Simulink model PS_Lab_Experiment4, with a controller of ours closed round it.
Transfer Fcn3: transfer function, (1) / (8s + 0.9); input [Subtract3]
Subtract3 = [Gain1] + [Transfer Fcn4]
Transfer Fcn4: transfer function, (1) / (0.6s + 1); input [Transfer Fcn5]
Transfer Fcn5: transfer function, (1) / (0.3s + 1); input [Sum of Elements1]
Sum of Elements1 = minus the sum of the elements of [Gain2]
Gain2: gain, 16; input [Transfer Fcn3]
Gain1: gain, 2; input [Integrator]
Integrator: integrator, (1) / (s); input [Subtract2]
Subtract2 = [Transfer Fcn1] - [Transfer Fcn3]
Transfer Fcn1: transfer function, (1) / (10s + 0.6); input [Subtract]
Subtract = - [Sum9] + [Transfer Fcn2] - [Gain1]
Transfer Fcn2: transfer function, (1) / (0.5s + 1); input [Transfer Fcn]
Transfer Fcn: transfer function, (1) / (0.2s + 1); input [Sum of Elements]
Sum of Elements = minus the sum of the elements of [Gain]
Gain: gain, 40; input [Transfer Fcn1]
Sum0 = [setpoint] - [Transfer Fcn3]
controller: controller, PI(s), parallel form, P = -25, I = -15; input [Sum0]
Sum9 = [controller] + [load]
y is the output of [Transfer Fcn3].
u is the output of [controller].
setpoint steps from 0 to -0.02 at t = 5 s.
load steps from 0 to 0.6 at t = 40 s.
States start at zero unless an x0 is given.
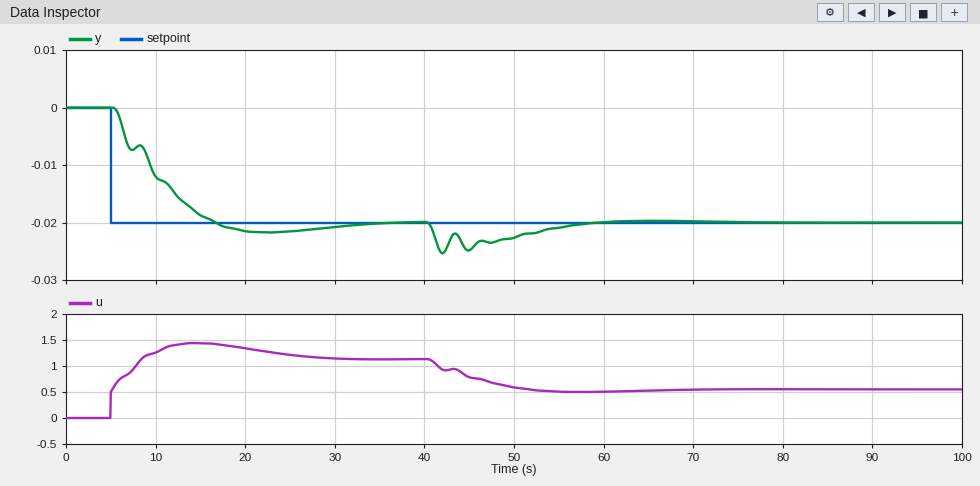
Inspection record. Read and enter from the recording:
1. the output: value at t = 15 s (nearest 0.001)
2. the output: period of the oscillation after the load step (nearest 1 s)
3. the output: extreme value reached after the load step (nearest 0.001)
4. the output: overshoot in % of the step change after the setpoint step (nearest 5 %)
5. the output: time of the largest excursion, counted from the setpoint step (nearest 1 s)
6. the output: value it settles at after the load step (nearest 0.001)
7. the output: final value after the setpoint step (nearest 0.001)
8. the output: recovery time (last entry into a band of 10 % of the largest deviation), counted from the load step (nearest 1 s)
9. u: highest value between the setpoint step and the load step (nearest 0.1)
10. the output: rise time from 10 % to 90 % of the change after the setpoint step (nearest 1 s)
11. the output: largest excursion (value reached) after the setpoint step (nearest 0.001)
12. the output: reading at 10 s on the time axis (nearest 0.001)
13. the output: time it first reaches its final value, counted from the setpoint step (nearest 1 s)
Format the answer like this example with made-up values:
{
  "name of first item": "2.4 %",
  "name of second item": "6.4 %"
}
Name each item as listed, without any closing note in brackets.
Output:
{
  "the output: value at t = 15 s": "-0.019",
  "the output: period of the oscillation after the load step": "3 s",
  "the output: extreme value reached after the load step": "-0.025",
  "the output: overshoot in % of the step change after the setpoint step": "10 %",
  "the output: time of the largest excursion, counted from the setpoint step": "18 s",
  "the output: value it settles at after the load step": "-0.020",
  "the output: final value after the setpoint step": "-0.020",
  "the output: recovery time (last entry into a band of 10 % of the largest deviation), counted from the load step": "16 s",
  "u: highest value between the setpoint step and the load step": "1.4",
  "the output: rise time from 10 % to 90 % of the change after the setpoint step": "8 s",
  "the output: largest excursion (value reached) after the setpoint step": "-0.022",
  "the output: reading at 10 s on the time axis": "-0.012",
  "the output: time it first reaches its final value, counted from the setpoint step": "12 s"
}
